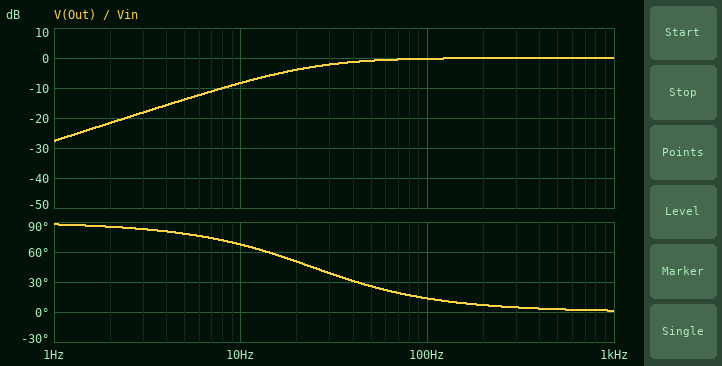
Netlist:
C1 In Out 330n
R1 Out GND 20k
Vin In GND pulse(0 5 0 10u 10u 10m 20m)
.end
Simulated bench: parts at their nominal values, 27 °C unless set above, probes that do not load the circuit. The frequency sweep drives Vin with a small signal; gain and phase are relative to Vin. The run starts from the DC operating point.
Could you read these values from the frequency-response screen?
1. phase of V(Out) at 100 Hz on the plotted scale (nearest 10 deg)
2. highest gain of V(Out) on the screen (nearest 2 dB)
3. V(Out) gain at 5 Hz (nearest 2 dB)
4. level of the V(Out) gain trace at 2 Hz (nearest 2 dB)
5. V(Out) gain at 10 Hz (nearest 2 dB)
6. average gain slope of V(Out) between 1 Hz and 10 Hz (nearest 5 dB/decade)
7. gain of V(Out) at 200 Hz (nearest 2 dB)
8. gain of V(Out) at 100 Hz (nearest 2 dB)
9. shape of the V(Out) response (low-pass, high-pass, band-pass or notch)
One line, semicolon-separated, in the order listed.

10 deg; 0 dB; -14 dB; -22 dB; -8 dB; 20 dB/decade; 0 dB; 0 dB; high-pass
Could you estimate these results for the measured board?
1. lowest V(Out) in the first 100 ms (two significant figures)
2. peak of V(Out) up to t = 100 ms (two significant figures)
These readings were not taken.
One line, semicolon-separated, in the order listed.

-4.1 V; 5.0 V
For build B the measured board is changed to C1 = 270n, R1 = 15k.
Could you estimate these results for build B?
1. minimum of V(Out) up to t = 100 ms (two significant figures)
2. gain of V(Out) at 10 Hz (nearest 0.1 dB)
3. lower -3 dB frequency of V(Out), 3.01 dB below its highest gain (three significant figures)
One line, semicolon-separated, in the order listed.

-4.6 V; -12.2 dB; 39.3 Hz
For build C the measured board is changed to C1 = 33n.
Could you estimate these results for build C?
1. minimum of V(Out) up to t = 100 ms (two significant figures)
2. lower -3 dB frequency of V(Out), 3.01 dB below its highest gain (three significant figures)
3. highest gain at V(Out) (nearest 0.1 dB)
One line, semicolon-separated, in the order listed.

-5.0 V; 241 Hz; 0 dB
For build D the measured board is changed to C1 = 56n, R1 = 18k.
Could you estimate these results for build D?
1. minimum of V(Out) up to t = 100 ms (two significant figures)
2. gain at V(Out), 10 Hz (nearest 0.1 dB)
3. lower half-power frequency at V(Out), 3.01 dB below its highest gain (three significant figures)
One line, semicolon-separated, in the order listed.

-5.0 V; -24.0 dB; 158 Hz
